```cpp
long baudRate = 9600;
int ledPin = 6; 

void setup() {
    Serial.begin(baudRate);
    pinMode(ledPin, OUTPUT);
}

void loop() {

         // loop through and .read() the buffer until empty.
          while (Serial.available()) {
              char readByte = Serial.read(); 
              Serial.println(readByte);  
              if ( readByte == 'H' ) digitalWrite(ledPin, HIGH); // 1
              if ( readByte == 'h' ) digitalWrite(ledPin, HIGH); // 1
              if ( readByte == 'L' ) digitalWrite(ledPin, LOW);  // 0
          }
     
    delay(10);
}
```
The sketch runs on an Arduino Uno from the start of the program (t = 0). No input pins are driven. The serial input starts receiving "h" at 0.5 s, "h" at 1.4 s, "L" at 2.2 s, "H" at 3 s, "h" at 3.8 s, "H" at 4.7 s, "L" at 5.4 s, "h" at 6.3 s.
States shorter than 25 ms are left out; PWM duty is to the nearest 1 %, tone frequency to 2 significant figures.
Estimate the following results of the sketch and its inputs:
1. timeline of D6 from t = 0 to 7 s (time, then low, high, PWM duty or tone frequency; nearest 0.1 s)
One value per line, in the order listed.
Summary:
0 s low; 0.5 s high; 2.2 s low; 3 s high; 5.4 s low; 6.3 s high
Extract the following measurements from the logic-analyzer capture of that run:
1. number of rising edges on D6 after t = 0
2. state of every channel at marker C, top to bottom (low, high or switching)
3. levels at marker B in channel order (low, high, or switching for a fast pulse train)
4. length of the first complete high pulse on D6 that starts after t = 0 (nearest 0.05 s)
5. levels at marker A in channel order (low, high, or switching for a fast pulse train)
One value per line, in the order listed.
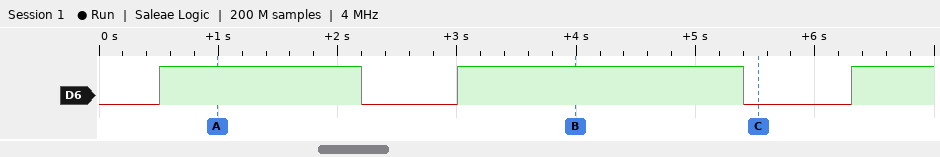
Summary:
3
D6 low
D6 high
1.70 s
D6 high
